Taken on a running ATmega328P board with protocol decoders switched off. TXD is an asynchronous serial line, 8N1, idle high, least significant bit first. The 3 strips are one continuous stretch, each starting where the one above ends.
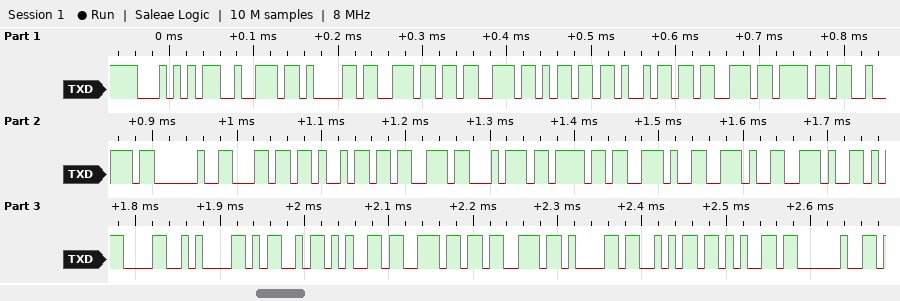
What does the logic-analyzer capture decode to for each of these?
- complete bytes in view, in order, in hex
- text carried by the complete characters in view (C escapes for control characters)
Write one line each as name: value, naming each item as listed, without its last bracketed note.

complete bytes in view, in order, in hex: 54 72 61 6E 73 6D 69 73 6F 72 20 6C 69 73 74 6F 2E 2E 2E 0D 0A 4D 65 6E 73 61 6A 65 20
text carried by the complete characters in view: "Transmisor listo...\r\nMensaje "
